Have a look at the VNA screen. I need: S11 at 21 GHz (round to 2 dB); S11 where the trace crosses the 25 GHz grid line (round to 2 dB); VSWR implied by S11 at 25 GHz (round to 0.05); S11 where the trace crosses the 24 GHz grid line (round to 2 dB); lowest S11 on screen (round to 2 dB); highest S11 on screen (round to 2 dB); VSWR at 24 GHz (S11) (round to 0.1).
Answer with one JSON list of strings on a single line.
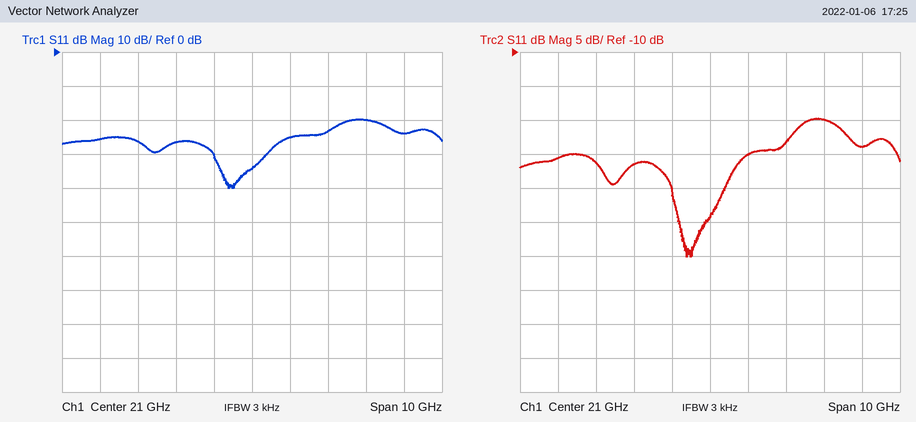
["-34 dB", "-24 dB", "1.15", "-20 dB", "-40 dB", "-20 dB", "1.2"]
